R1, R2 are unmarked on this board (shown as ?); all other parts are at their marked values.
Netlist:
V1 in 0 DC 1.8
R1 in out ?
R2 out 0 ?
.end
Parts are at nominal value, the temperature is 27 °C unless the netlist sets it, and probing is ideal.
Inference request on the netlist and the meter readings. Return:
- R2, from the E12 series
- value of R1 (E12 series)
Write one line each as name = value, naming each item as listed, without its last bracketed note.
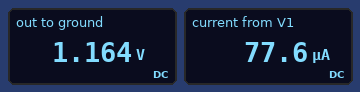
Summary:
R2, from the E12 series = 15 kΩ
value of R1 = 8.2 kΩ
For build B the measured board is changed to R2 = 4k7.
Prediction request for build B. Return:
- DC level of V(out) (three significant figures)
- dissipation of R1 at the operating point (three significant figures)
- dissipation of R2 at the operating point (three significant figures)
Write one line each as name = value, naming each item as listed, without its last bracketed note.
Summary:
DC level of V(out) = 656 mV
dissipation of R1 at the operating point = 160 µW
dissipation of R2 at the operating point = 91.5 µW
